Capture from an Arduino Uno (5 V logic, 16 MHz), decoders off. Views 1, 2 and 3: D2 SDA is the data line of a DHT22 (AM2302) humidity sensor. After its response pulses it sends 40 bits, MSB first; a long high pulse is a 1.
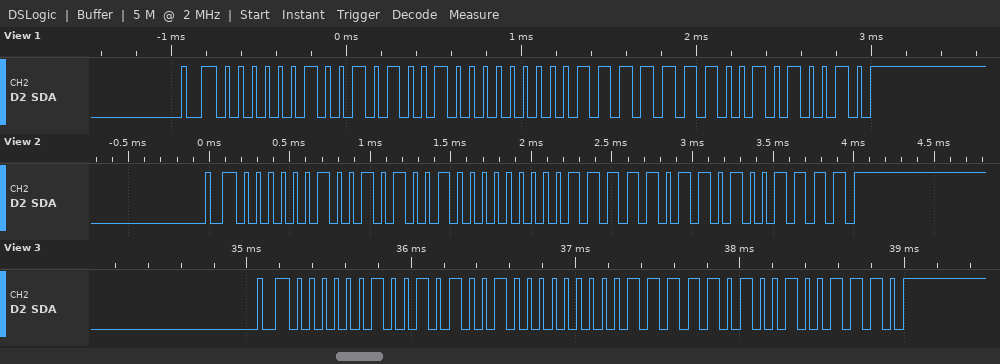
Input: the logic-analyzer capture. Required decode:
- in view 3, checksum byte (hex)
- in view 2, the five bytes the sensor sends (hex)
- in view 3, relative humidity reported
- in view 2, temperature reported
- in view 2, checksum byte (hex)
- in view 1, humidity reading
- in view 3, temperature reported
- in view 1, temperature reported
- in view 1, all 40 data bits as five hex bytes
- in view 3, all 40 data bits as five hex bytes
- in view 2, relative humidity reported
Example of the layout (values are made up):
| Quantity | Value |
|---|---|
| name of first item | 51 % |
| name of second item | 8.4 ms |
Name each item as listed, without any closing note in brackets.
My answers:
| Quantity | Value |
|---|---|
| in view 3, checksum byte | 0x4E |
| in view 2, the five bytes the sensor sends | 02 52 00 FB 4F |
| in view 3, relative humidity reported | 59.4 % |
| in view 2, temperature reported | 25.1 °C |
| in view 2, checksum byte | 0x4F |
| in view 1, humidity reading | 59.4 % |
| in view 3, temperature reported | 25.0 °C |
| in view 1, temperature reported | 25.4 °C |
| in view 1, all 40 data bits as five hex bytes | 02 52 00 FE 52 |
| in view 3, all 40 data bits as five hex bytes | 02 52 00 FA 4E |
| in view 2, relative humidity reported | 59.4 % |
